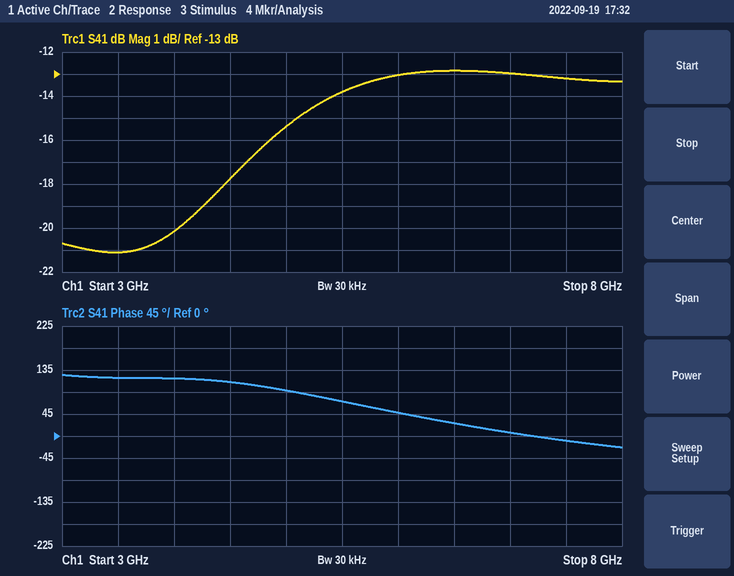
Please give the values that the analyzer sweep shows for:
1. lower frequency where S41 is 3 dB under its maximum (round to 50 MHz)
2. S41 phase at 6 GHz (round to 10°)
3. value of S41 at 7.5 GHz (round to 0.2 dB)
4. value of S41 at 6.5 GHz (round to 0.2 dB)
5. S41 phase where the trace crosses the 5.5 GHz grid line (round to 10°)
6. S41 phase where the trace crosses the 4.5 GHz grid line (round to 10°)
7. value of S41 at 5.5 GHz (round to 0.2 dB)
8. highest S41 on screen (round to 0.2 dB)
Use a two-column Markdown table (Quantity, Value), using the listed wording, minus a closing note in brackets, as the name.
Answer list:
| Quantity | Value |
|---|---|
| lower frequency where S41 is 3 dB under its maximum | 4.90 GHz |
| S41 phase at 6 GHz | 50° |
| value of S41 at 7.5 GHz | -13.2 dB |
| value of S41 at 6.5 GHz | -12.8 dB |
| S41 phase where the trace crosses the 5.5 GHz grid line | 70° |
| S41 phase where the trace crosses the 4.5 GHz grid line | 110° |
| value of S41 at 5.5 GHz | -13.8 dB |
| highest S41 on screen | -12.8 dB |
